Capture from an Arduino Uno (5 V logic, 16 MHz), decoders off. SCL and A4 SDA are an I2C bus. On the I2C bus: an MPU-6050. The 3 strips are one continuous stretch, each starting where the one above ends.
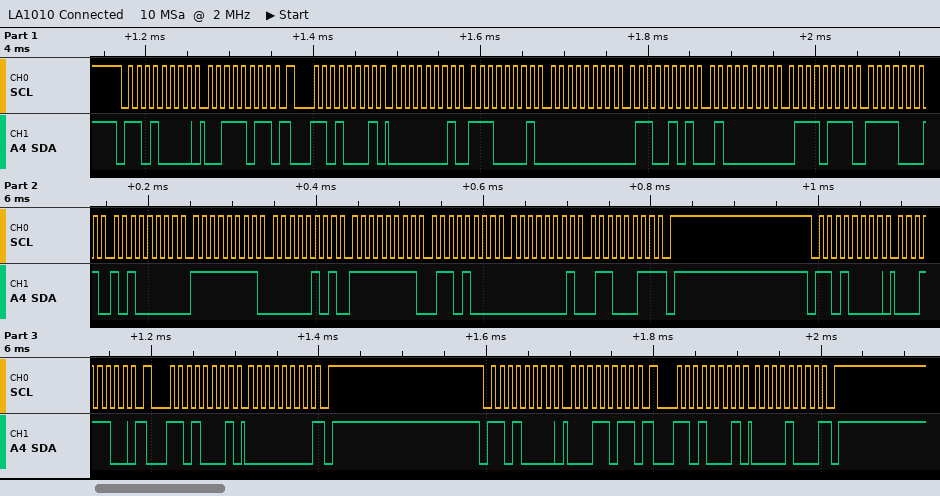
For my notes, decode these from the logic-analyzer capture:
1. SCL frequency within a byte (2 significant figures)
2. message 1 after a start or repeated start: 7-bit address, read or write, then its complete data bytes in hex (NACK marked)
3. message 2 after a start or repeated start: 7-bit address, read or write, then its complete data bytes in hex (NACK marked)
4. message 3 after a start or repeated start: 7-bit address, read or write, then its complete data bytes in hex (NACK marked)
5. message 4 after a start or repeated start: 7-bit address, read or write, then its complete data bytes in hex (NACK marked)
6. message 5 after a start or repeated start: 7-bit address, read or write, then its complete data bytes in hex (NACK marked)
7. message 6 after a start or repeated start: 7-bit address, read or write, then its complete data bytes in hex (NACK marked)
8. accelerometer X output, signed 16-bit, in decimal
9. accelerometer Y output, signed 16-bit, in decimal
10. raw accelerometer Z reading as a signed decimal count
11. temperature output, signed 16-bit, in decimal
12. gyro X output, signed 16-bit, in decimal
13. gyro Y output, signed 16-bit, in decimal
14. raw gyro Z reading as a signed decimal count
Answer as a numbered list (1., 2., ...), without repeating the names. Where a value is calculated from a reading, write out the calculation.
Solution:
1. 100 kHz
2. 0x68 write: 3B
3. 0x68 read: 01 E1 00 65 40 77 F1 A0 FF 05 FF 68 01 63 NACK
4. 0x68 write: 1C
5. 0x68 read: 00 NACK
6. 0x68 write: 1B
7. 0x68 read: 08 NACK
8. 0x01E1 = 481
9. 0x0065 = 101
10. 0x4077 = 16503
11. 0xF1A0 = -3680
12. 0xFF05 = -251
13. 0xFF68 = -152
14. 0x0163 = 355
